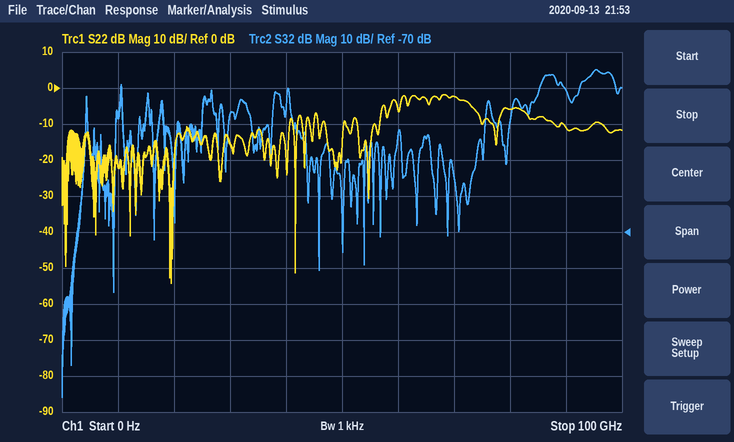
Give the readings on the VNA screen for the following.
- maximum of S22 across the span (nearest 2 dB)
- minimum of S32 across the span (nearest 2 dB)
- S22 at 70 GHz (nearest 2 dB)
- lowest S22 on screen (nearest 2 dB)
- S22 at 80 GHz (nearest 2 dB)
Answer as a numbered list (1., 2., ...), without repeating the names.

1. -2 dB
2. -116 dB
3. -2 dB
4. -54 dB
5. -6 dB
